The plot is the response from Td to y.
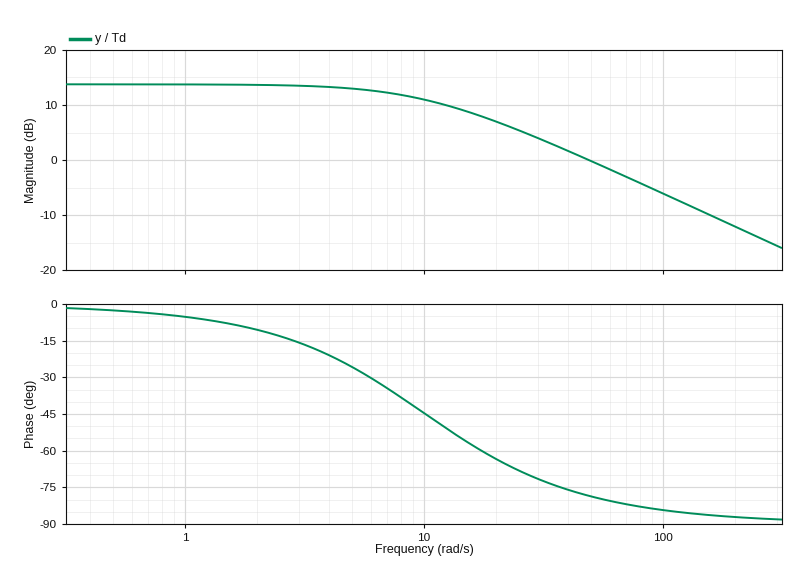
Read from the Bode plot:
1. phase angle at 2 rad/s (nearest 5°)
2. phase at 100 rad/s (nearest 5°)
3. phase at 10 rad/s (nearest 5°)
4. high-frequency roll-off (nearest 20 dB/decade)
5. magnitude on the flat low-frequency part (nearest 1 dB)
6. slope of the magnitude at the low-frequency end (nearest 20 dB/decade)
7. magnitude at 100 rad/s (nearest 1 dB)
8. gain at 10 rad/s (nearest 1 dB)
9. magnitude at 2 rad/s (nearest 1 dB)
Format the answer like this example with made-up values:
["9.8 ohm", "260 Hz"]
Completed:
["-10°", "-85°", "-45°", "-20 dB/decade", "14 dB", "0 dB/decade", "-6 dB", "11 dB", "14 dB"]
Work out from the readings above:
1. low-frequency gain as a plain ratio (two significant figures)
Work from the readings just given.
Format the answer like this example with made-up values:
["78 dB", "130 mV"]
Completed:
["5.0"]
